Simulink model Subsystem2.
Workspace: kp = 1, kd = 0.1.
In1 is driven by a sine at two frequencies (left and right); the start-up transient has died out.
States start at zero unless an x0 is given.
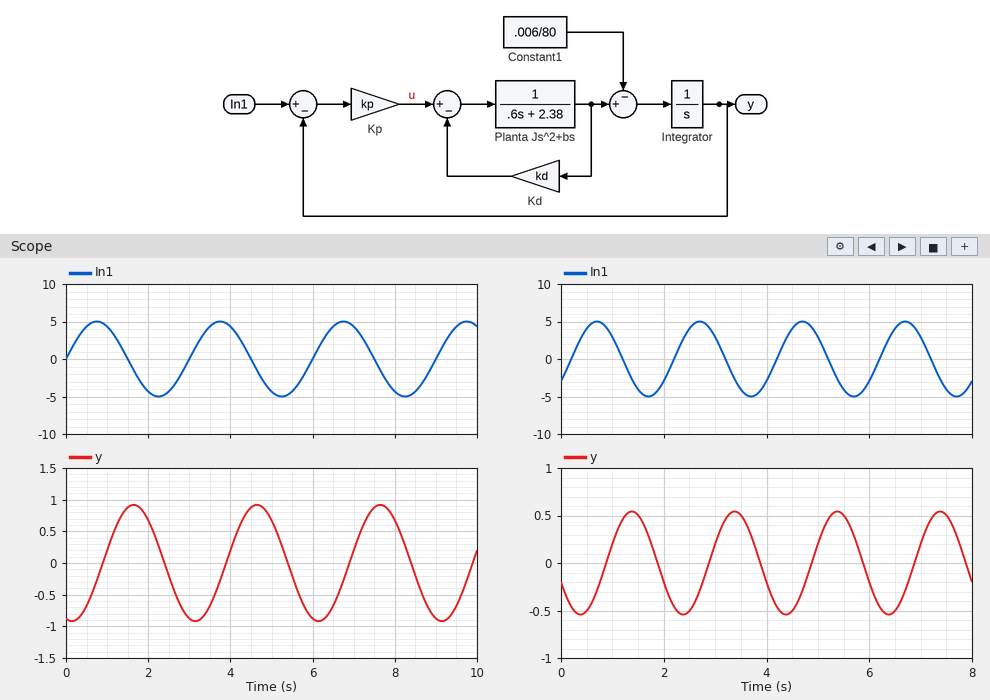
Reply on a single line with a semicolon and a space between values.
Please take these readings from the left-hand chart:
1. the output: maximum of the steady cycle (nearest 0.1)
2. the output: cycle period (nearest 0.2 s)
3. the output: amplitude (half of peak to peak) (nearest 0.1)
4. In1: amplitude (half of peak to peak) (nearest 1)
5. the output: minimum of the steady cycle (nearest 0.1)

0.9; 3.0 s; 0.9; 5; -0.9
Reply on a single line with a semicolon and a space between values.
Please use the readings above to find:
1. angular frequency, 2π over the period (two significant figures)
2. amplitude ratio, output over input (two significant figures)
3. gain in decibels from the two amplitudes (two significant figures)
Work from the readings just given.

2.1 rad/s; 0.18; -15 dB
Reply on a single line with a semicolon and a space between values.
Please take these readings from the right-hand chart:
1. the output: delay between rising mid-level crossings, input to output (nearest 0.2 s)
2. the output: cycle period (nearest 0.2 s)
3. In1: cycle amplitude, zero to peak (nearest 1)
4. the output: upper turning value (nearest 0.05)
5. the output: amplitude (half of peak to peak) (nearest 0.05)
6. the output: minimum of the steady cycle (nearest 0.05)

0.6 s; 2.0 s; 5; 0.55; 0.55; -0.55
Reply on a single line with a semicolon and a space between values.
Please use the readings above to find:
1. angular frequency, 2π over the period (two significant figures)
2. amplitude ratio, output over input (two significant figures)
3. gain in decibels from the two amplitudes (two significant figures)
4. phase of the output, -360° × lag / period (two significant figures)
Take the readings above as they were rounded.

3.1 rad/s; 0.11; -19 dB; -110°
